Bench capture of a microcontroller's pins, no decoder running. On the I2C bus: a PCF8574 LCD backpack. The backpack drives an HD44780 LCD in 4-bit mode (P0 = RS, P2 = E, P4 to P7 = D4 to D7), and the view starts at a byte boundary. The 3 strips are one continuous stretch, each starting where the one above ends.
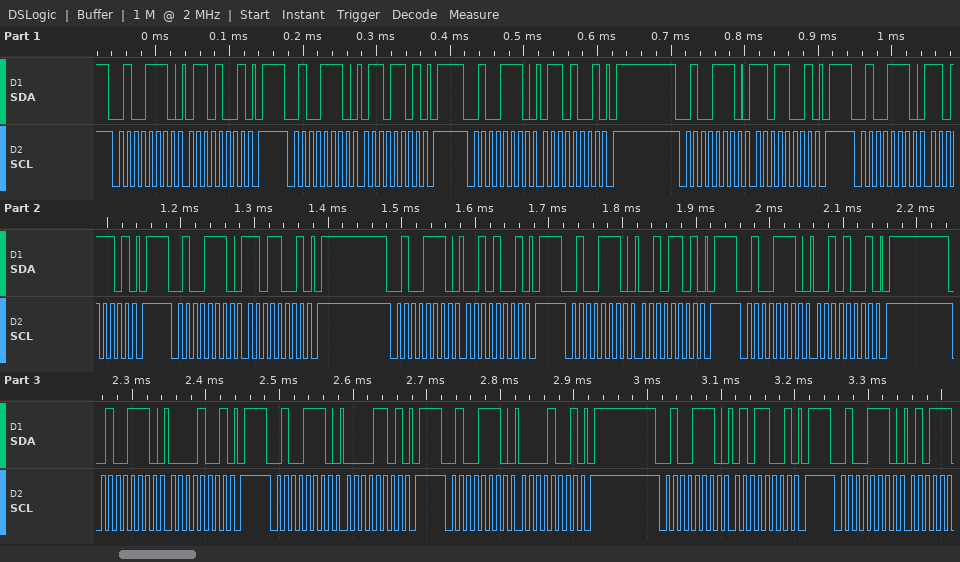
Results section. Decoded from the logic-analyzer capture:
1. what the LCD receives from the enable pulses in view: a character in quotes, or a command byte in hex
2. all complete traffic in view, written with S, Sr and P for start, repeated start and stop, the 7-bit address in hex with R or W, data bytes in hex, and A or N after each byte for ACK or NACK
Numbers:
'm' ' '
S 27W A 69 A P S 27W A 6D A P S 27W A 69 A P S 27W A D9 A P S 27W A DD A P S 27W A D9 A P S 27W A 29 A P S 27W A 2D A P S 27W A 29 A P S 27W A 09 A P S 27W A 0D A P S 27W A 09 A P S 27W A 59 A P S 27W A
